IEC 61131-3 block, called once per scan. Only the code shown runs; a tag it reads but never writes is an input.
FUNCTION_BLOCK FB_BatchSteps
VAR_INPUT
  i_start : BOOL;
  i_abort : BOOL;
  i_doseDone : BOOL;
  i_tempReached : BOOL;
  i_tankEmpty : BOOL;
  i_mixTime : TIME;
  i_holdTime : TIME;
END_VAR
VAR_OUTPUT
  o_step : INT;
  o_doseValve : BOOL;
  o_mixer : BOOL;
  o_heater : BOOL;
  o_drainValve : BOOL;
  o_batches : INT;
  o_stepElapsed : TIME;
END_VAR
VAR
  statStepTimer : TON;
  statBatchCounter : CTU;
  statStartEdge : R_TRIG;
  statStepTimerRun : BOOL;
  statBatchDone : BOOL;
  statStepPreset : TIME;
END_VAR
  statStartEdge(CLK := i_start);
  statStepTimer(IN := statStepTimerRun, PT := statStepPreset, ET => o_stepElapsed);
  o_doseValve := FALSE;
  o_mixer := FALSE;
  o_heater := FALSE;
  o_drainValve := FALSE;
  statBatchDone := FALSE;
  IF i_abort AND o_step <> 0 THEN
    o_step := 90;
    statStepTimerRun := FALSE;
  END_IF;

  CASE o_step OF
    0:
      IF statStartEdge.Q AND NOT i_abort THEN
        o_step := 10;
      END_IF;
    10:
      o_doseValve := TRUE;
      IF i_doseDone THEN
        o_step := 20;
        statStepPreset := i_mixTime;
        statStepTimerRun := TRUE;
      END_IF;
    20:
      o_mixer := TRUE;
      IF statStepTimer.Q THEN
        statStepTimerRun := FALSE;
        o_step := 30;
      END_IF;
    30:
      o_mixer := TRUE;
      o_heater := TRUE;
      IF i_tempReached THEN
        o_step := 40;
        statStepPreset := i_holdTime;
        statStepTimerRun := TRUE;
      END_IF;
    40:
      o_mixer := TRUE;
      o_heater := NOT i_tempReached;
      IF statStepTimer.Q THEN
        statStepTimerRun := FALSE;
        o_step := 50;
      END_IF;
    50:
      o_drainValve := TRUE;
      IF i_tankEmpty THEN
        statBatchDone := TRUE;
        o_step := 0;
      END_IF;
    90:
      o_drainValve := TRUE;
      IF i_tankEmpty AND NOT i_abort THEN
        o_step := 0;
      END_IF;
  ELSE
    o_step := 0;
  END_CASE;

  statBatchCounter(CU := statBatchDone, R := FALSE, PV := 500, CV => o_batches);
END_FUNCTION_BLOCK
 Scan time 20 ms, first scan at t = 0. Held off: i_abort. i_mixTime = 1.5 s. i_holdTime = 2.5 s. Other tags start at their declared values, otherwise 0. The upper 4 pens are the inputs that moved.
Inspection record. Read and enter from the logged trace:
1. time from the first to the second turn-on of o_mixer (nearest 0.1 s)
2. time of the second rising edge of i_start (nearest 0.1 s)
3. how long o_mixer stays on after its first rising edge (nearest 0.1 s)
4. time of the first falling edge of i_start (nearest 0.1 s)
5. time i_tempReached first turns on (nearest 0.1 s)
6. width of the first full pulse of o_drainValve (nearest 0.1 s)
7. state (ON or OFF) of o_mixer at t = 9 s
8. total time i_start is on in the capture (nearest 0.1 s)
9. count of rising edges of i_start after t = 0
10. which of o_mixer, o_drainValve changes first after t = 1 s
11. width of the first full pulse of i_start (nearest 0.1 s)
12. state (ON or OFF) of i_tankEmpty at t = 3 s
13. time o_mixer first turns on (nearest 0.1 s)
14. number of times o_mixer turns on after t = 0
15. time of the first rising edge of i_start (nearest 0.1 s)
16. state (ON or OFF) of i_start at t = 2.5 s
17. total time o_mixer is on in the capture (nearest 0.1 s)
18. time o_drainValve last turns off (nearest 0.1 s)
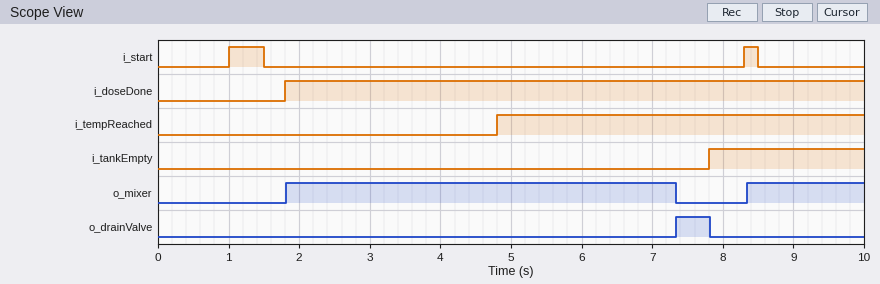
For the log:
6.5 s
8.3 s
5.5 s
1.5 s
4.8 s
0.5 s
ON
0.7 s
2
o_mixer
0.5 s
OFF
1.8 s
2
1.0 s
OFF
7.2 s
7.8 s
